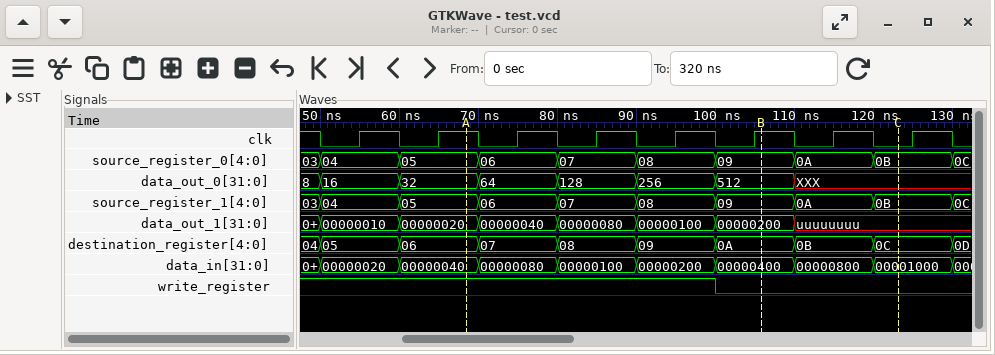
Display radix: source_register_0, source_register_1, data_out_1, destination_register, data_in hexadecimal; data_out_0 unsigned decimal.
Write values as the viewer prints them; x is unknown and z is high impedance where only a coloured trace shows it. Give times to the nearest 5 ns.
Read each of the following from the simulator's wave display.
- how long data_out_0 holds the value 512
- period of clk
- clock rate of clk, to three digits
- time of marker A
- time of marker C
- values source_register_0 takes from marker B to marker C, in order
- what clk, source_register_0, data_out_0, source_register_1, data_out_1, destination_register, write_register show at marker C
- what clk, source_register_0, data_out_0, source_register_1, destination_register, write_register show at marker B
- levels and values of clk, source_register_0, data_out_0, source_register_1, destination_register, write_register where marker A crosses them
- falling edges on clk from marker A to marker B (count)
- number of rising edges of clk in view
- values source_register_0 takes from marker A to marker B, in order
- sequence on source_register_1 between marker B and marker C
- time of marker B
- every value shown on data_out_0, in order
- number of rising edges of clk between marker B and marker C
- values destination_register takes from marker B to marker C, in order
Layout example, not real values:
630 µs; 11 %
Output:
10 ns; 10 ns; 100 MHz; 70 ns; 125 ns; 09, 0A, 0B; clk=0, source_register_0=0B, data_out_0=XXX, source_register_1=0B, data_out_1=uuuuuuuu, destination_register=0C, write_register=0; clk=1, source_register_0=09, data_out_0=512, source_register_1=09, destination_register=0A, write_register=0; clk=1, source_register_0=05, data_out_0=32, source_register_1=05, destination_register=06, write_register=1; 4; 8; 05, 06, 07, 08, 09; 09, 0A, 0B; 105 ns; 8, 16, 32, 64, 128, 256, 512, XXX; 1; 0A, 0B, 0C
